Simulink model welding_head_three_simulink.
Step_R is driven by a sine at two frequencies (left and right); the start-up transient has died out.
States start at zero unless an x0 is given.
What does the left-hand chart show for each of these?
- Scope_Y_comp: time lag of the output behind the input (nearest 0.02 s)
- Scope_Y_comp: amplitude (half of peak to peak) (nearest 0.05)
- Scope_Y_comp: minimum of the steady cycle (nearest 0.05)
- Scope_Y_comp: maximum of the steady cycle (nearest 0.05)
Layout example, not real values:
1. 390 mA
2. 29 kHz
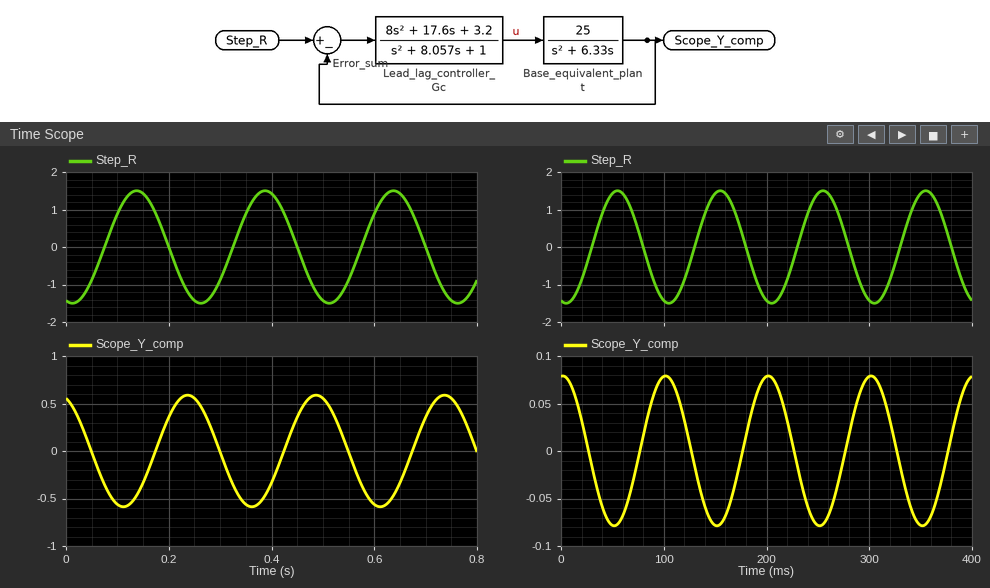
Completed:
1. 0.10 s
2. 0.60
3. -0.60
4. 0.60
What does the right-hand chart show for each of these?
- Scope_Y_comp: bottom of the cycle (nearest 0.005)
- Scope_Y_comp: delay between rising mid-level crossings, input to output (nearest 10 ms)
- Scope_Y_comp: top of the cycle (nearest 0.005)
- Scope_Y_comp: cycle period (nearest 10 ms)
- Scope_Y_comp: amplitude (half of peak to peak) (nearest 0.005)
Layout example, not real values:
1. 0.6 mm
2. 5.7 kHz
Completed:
1. -0.080
2. 50 ms
3. 0.080
4. 100 ms
5. 0.080
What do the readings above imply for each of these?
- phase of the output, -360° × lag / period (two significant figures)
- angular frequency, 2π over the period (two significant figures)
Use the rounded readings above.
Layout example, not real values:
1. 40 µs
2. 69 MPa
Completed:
1. -180°
2. 0.063 rad/ms
